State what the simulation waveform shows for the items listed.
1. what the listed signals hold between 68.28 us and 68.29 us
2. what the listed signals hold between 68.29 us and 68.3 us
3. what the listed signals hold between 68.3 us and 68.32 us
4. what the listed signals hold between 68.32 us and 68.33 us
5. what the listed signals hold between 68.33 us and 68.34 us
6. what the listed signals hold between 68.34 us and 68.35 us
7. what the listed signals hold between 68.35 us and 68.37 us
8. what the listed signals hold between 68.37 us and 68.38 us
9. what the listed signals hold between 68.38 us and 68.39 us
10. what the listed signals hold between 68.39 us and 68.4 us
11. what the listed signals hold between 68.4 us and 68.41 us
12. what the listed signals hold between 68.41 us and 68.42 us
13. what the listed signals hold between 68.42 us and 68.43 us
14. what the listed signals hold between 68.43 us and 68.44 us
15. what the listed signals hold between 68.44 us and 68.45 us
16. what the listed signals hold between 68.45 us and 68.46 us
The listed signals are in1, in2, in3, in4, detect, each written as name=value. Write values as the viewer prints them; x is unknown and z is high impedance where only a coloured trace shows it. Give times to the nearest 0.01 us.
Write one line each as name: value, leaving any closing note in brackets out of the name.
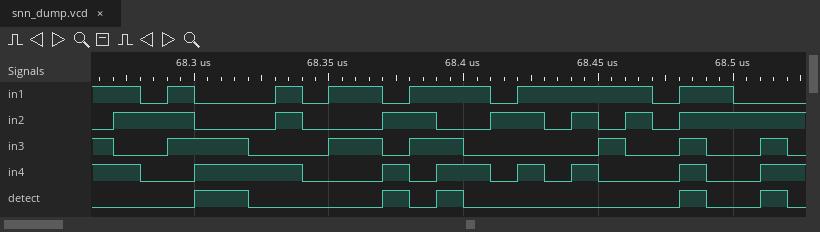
what the listed signals hold between 68.28 us and 68.29 us: in1=0, in2=1, in3=0, in4=0, detect=0
what the listed signals hold between 68.29 us and 68.3 us: in1=1, in2=1, in3=1, in4=0, detect=0
what the listed signals hold between 68.3 us and 68.32 us: in1=0, in2=0, in3=1, in4=1, detect=1
what the listed signals hold between 68.32 us and 68.33 us: in1=0, in2=0, in3=0, in4=1, detect=0
what the listed signals hold between 68.33 us and 68.34 us: in1=1, in2=1, in3=0, in4=1, detect=0
what the listed signals hold between 68.34 us and 68.35 us: in1=0, in2=0, in3=0, in4=0, detect=0
what the listed signals hold between 68.35 us and 68.37 us: in1=1, in2=0, in3=1, in4=0, detect=0
what the listed signals hold between 68.37 us and 68.38 us: in1=0, in2=1, in3=0, in4=1, detect=1
what the listed signals hold between 68.38 us and 68.39 us: in1=1, in2=1, in3=1, in4=0, detect=0
what the listed signals hold between 68.39 us and 68.4 us: in1=1, in2=0, in3=1, in4=1, detect=1
what the listed signals hold between 68.4 us and 68.41 us: in1=1, in2=0, in3=0, in4=1, detect=0
what the listed signals hold between 68.41 us and 68.42 us: in1=0, in2=1, in3=0, in4=0, detect=0
what the listed signals hold between 68.42 us and 68.43 us: in1=1, in2=1, in3=0, in4=1, detect=0
what the listed signals hold between 68.43 us and 68.44 us: in1=1, in2=0, in3=0, in4=0, detect=0
what the listed signals hold between 68.44 us and 68.45 us: in1=1, in2=1, in3=0, in4=1, detect=0
what the listed signals hold between 68.45 us and 68.46 us: in1=1, in2=0, in3=1, in4=0, detect=0
